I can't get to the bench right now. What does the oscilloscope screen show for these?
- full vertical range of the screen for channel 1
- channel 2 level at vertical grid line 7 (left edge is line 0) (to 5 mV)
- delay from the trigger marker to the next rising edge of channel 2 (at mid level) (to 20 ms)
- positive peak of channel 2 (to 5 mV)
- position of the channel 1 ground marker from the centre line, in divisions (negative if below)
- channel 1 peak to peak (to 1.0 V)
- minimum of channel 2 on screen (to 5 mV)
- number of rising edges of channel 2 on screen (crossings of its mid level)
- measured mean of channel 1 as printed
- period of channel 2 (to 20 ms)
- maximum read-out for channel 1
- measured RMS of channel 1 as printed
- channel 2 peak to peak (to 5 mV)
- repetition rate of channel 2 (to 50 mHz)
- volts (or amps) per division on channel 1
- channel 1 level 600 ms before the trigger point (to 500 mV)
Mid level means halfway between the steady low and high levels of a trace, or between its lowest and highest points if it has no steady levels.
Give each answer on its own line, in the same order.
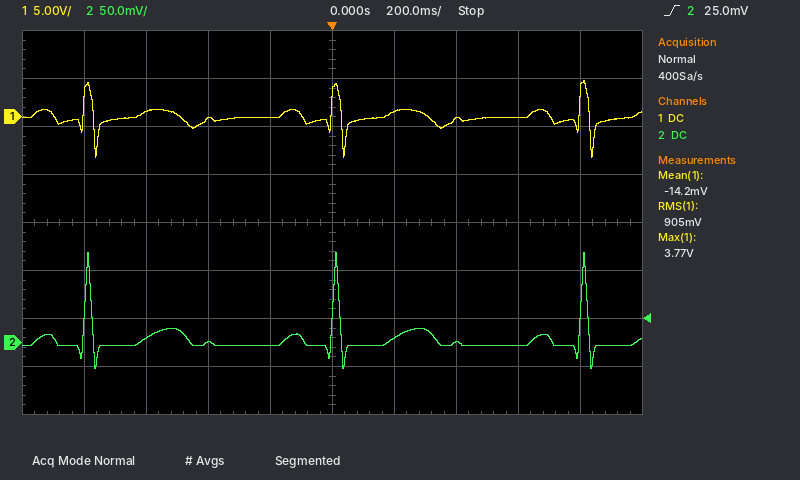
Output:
40 V
0 mV
800 ms
95 mV
+2.2 div
8.0 V
-25 mV
3
-14.2 mV
800 ms
3.77 V
905 mV
120 mV
1.25 Hz
5 V
500 mV
